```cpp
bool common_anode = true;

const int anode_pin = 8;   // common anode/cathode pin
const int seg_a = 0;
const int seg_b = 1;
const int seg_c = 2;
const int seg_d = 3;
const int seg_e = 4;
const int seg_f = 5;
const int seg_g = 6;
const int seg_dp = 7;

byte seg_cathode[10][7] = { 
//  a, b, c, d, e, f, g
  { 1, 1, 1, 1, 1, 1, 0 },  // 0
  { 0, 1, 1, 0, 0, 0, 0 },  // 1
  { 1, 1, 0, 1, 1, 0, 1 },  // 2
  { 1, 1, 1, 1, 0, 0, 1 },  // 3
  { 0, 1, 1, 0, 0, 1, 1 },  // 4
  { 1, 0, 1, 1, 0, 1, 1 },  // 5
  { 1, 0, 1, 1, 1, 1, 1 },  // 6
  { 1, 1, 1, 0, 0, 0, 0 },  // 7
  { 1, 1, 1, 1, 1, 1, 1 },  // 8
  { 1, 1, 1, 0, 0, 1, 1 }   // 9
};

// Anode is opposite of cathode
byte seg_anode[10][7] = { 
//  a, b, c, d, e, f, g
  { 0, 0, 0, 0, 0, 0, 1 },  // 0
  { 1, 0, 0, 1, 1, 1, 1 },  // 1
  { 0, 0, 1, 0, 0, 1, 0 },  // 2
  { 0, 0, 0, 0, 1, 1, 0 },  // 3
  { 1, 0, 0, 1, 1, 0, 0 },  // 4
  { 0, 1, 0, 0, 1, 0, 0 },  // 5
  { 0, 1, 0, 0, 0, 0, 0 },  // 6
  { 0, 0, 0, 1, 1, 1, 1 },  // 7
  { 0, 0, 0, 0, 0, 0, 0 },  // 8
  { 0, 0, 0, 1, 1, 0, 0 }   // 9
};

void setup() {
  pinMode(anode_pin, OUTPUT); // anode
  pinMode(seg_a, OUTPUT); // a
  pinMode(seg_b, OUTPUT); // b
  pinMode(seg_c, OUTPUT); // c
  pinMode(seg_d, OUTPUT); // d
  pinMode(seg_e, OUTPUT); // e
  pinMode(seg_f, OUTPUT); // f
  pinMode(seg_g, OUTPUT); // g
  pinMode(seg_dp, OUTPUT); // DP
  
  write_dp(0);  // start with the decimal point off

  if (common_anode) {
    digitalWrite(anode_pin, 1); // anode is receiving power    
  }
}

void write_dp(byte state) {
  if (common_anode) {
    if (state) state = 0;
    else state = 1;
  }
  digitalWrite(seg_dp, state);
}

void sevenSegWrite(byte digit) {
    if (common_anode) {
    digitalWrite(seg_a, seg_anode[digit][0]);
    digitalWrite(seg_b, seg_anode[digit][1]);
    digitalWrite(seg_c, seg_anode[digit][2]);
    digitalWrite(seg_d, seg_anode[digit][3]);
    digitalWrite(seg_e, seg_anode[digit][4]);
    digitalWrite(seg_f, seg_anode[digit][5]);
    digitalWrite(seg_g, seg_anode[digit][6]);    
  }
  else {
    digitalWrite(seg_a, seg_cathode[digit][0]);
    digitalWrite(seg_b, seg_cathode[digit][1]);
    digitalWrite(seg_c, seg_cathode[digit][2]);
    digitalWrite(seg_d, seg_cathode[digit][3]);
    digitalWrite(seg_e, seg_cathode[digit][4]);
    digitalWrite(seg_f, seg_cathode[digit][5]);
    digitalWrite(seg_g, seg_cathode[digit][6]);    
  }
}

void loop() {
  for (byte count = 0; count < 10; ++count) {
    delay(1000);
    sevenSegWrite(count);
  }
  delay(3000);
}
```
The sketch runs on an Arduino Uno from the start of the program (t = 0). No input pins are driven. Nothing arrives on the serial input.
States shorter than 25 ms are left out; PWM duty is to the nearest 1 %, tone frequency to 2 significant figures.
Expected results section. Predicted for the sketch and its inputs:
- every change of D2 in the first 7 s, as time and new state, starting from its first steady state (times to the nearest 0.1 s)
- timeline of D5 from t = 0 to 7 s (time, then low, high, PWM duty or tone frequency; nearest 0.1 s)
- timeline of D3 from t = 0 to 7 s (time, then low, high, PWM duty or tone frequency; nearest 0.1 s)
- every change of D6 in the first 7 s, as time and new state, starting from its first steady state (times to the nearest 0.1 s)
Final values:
0 s low; 3 s high; 4 s low
0 s low; 2 s high; 5 s low
0 s low; 2 s high; 3 s low; 5 s high; 6 s low
0 s low; 1 s high; 3 s low
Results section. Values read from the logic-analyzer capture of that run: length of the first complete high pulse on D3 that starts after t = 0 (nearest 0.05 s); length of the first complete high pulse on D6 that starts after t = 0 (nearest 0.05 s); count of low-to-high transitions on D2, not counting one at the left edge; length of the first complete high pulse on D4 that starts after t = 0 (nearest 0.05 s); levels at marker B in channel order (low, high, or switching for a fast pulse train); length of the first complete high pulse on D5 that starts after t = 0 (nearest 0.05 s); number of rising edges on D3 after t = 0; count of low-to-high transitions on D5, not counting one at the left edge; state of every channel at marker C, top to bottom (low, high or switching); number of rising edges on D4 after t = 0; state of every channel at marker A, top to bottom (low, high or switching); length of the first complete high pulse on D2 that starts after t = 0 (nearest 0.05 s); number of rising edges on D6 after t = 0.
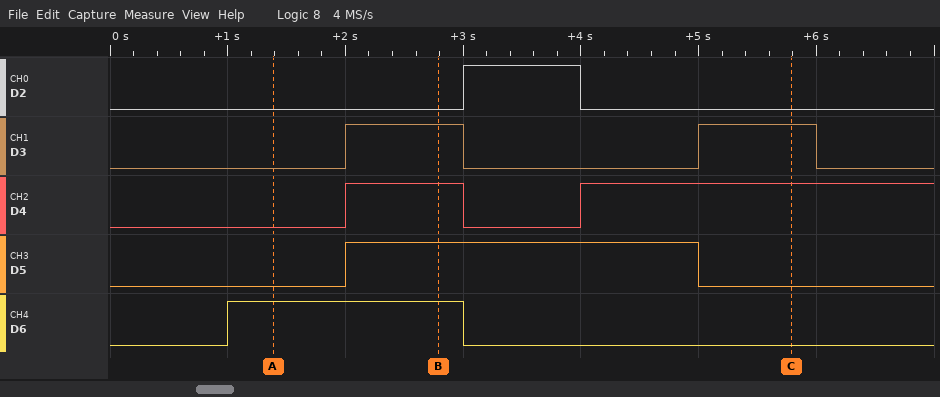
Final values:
1.00 s
2.00 s
1
1.00 s
D2 low, D3 high, D4 high, D5 high, D6 high
3.00 s
2
1
D2 low, D3 high, D4 high, D5 low, D6 low
2
D2 low, D3 low, D4 low, D5 low, D6 high
1.00 s
1
